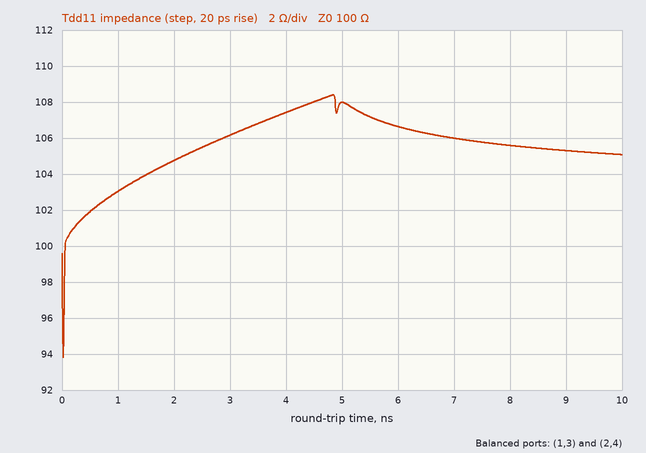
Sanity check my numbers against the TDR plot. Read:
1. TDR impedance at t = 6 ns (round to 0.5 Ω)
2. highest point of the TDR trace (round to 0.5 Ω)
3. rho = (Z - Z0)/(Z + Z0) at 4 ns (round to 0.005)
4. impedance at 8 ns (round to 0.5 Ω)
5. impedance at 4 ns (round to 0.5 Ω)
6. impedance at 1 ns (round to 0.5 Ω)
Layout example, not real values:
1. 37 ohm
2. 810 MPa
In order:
1. 106.5 Ω
2. 108.5 Ω
3. +0.035
4. 105.5 Ω
5. 107.5 Ω
6. 103.0 Ω
